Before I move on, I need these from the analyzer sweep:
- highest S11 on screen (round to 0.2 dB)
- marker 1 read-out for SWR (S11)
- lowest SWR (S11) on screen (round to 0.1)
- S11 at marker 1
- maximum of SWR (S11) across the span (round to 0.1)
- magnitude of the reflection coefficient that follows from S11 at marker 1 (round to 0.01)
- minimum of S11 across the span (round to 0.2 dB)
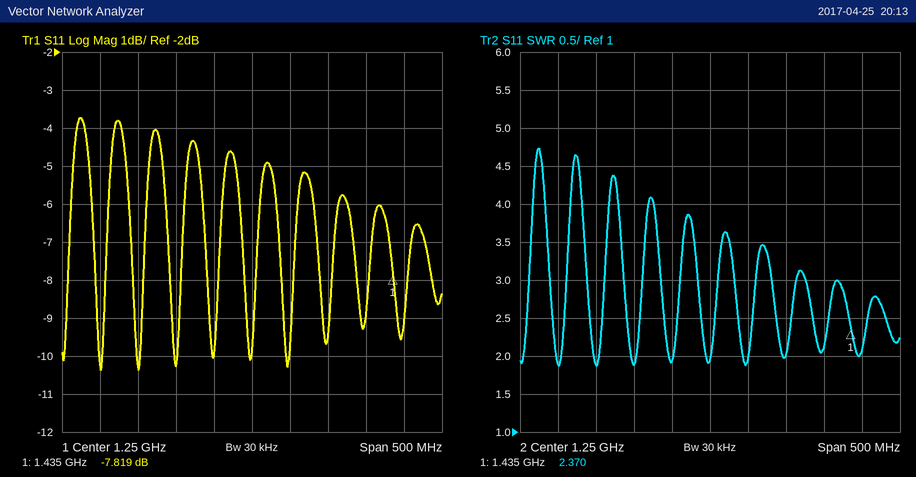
-3.8 dB
2.370
1.9
-7.819 dB
4.7
0.41
-10.4 dB
